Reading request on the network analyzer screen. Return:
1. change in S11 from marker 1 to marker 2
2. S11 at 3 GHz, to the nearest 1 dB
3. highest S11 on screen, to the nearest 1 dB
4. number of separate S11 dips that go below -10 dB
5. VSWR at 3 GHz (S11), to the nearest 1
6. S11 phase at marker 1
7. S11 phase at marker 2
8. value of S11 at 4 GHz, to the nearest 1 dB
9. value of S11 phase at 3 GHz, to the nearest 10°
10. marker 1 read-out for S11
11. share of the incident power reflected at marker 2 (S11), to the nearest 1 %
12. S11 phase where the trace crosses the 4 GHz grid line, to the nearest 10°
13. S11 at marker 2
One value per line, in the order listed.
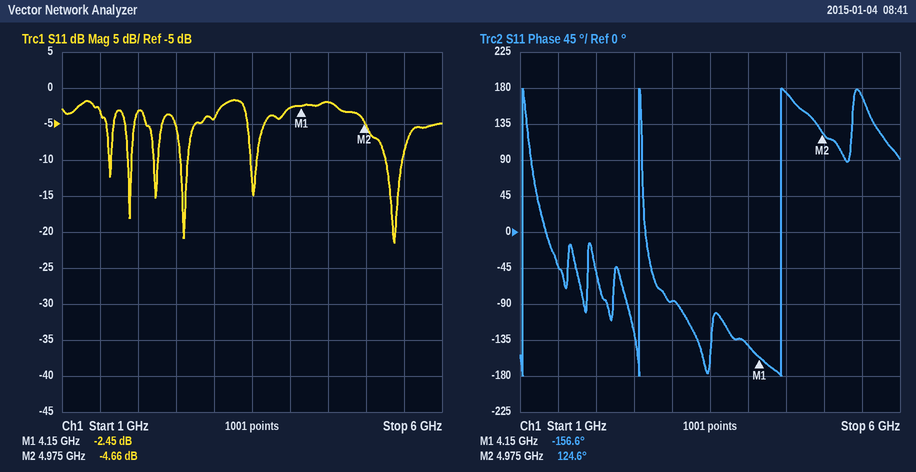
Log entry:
-2.21 dB
-4 dB
-2 dB
6
4
-156.6°
124.6°
-3 dB
-90°
-2.45 dB
34 %
-140°
-4.66 dB
